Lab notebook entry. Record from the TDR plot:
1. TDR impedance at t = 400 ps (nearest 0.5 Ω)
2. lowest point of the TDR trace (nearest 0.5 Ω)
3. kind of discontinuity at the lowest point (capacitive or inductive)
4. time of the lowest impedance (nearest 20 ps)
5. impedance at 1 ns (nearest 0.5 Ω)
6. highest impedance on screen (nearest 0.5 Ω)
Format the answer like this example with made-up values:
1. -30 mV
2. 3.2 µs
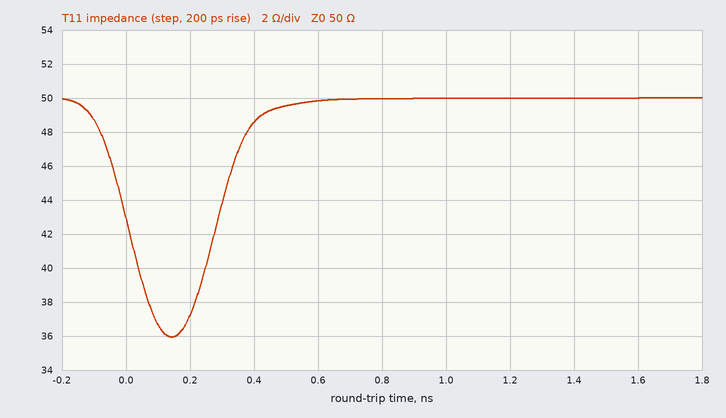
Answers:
1. 48.5 Ω
2. 36.0 Ω
3. capacitive
4. 140 ps
5. 50.0 Ω
6. 50.0 Ω
